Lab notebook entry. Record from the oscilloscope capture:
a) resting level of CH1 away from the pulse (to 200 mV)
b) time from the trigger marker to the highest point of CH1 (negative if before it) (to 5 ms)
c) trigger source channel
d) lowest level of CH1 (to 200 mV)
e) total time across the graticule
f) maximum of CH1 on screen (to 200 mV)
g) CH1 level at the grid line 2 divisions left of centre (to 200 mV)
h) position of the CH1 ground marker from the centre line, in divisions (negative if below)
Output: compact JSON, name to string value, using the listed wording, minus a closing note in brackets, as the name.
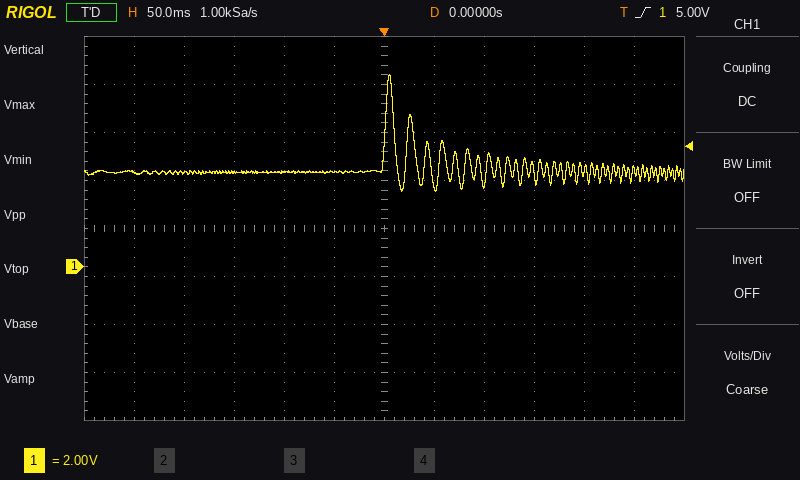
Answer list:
{"resting level of CH1 away from the pulse": "4.0 V", "time from the trigger marker to the highest point of CH1 (negative if before it)": "+5 ms", "trigger source channel": "CH1", "lowest level of CH1": "3.2 V", "total time across the graticule": "600 ms", "maximum of CH1 on screen": "8.0 V", "CH1 level at the grid line 2 divisions left of centre": "4.0 V", "position of the CH1 ground marker from the centre line, in divisions": "-0.8 div"}
